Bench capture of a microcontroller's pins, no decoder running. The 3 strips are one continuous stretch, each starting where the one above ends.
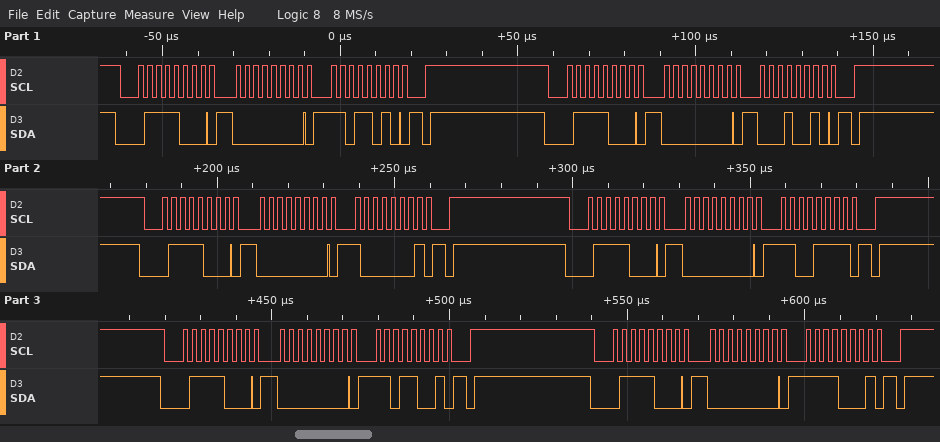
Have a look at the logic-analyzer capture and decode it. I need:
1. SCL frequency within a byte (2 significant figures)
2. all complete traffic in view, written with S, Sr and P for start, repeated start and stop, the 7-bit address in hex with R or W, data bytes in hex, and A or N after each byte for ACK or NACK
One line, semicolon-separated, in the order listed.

400 kHz; S 3CW A 00 A DA A P S 3CW A 00 A 12 A P S 3CW A 00 A 81 A P S 3CW A 00 A CF A P S 3CW A 00 A D9 A P S 3CW A 00 A F1 A P
